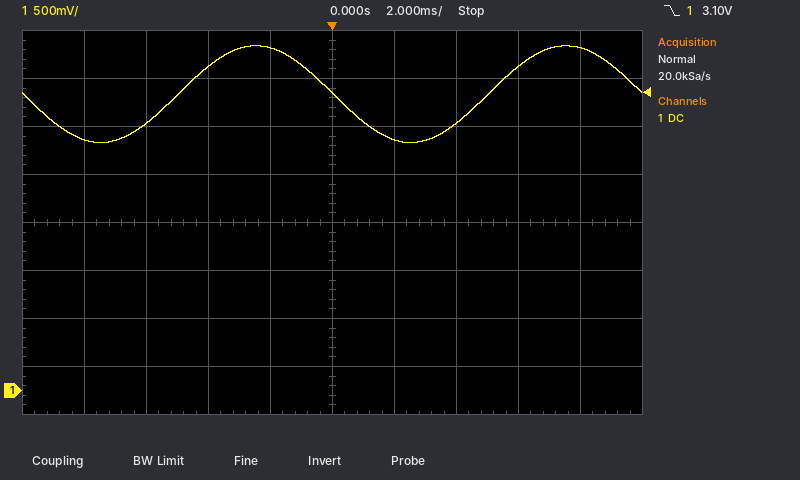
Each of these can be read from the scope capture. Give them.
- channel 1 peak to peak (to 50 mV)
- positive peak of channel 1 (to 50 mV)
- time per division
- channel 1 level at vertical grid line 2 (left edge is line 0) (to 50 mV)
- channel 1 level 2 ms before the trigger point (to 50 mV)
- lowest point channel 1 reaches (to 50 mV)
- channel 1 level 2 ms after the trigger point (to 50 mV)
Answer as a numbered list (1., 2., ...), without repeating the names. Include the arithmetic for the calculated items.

1. 3.60 V − (2.60 V) = 1.00 V
2. 3.60 V
3. 2 ms
4. 2.80 V
5. 3.55 V
6. 2.60 V
7. 2.60 V
